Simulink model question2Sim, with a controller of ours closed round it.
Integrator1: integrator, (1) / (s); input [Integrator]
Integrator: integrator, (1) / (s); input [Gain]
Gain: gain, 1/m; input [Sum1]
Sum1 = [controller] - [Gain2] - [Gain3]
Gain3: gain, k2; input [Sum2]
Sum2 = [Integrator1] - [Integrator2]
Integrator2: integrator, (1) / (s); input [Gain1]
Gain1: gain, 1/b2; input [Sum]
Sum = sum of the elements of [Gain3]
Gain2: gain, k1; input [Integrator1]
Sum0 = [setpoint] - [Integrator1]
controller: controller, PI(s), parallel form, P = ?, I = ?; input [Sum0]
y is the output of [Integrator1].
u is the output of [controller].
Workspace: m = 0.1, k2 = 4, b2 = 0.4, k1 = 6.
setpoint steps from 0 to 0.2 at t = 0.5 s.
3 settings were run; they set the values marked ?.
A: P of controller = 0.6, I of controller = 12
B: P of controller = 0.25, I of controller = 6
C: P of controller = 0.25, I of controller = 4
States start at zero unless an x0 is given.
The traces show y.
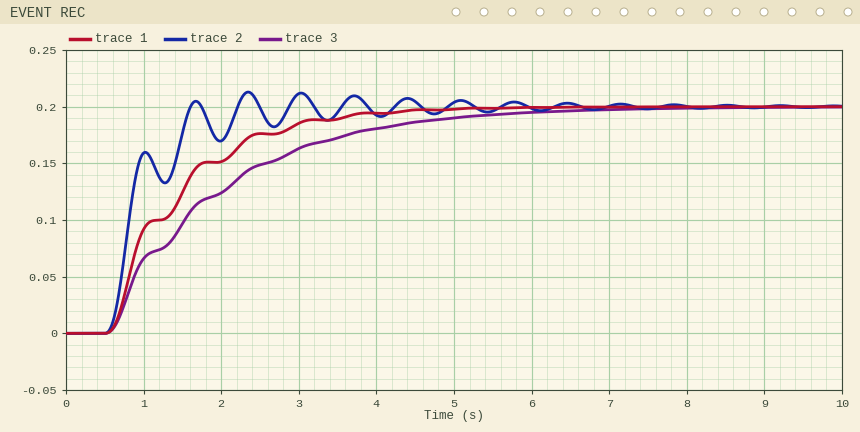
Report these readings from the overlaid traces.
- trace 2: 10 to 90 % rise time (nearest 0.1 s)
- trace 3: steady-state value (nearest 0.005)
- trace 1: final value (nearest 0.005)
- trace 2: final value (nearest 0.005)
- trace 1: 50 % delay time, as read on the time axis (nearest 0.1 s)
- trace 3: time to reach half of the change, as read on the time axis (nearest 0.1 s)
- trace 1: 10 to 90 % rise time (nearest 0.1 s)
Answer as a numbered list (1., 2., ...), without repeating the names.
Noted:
1. 0.9 s
2. 0.200
3. 0.200
4. 0.200
5. 1.2 s
6. 1.5 s
7. 2.2 s
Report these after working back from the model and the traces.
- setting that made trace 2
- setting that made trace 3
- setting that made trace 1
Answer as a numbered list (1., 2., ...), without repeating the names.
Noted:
1. A
2. C
3. B
